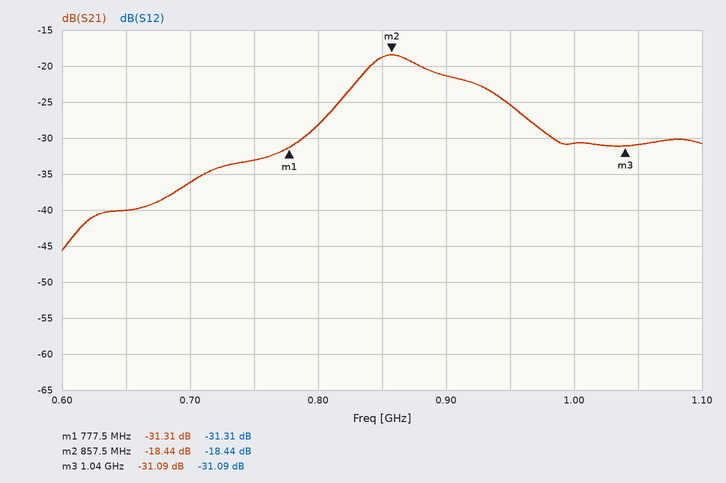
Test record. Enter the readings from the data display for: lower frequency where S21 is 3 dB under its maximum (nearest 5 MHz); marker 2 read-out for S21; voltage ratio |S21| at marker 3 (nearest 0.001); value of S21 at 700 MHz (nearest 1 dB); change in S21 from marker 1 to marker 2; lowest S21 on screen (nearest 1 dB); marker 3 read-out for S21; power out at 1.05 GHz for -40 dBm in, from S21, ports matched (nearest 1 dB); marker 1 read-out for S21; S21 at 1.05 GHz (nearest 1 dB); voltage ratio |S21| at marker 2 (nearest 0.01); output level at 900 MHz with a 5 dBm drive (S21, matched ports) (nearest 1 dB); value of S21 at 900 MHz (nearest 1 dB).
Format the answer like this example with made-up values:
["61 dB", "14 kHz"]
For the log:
["835 MHz", "-18.44 dB", "0.028", "-36 dB", "12.87 dB", "-46 dB", "-31.09 dB", "-71 dBm", "-31.31 dB", "-31 dB", "0.12", "-16 dBm", "-21 dB"]
